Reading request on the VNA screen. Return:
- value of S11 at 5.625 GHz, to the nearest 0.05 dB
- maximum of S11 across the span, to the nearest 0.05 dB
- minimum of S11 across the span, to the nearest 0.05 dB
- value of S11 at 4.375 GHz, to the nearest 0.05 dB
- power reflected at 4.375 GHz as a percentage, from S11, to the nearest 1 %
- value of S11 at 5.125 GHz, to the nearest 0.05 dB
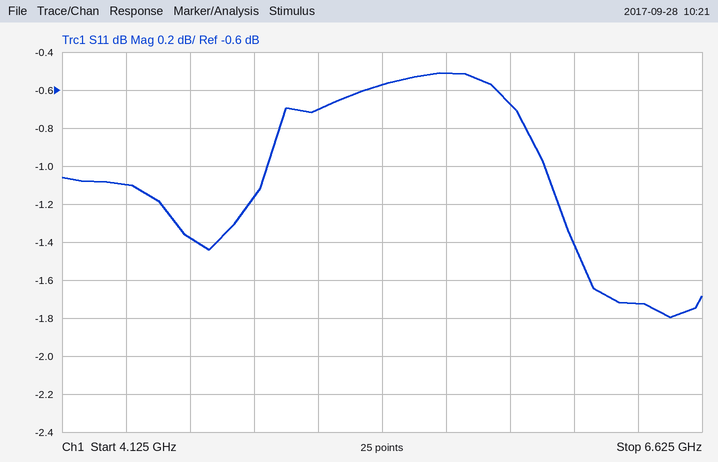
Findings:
-0.50 dB
-0.50 dB
-1.80 dB
-1.10 dB
78 %
-0.70 dB
